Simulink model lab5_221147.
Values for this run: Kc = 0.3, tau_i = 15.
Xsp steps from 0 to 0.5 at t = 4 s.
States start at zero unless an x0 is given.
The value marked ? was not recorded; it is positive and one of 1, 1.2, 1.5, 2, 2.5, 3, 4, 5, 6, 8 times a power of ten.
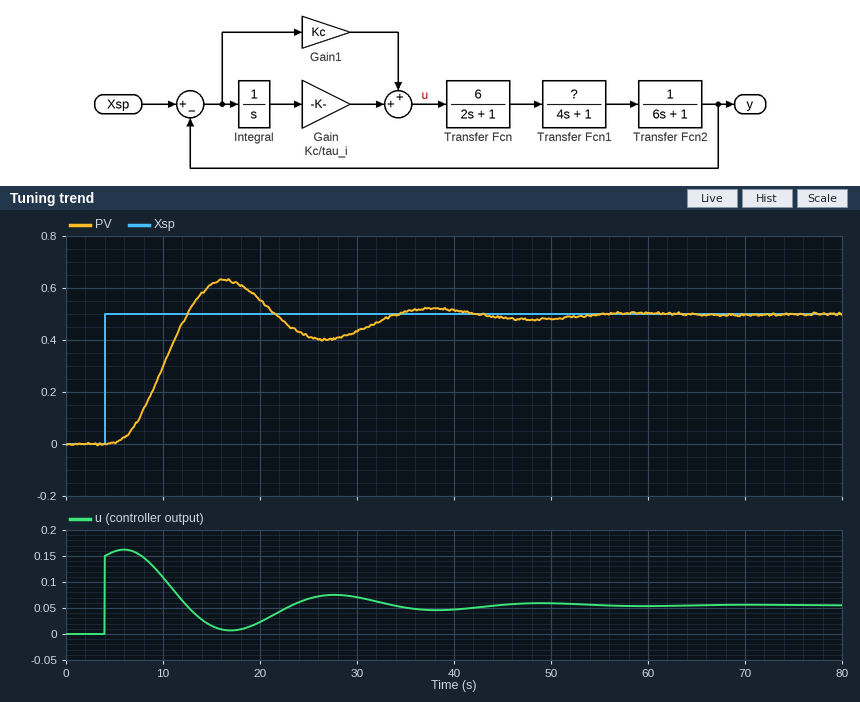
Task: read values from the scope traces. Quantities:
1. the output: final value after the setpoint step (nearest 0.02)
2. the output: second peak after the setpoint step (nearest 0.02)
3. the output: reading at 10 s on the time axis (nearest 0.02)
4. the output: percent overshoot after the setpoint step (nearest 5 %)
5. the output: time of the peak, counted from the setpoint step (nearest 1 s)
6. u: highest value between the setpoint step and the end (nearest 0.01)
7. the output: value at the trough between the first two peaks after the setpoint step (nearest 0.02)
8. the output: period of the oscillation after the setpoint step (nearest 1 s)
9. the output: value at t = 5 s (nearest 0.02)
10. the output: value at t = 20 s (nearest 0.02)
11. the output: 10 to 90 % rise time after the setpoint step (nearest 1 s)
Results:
0.50
0.52
0.30
25 %
12 s
0.16
0.40
21 s
0.00
0.56
5 s
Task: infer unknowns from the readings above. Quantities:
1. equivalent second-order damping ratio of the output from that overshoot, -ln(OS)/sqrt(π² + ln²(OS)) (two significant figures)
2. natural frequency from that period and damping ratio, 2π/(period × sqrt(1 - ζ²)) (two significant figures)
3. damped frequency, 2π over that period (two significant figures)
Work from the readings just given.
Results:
0.40
0.33 rad/s
0.30 rad/s
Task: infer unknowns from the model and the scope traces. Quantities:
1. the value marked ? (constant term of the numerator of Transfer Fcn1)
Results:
1.5
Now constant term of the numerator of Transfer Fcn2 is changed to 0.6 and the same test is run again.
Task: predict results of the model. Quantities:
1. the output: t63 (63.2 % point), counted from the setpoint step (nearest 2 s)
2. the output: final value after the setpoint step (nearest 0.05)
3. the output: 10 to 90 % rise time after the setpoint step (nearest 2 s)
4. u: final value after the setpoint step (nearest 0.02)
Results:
8 s
0.50
8 s
0.10
